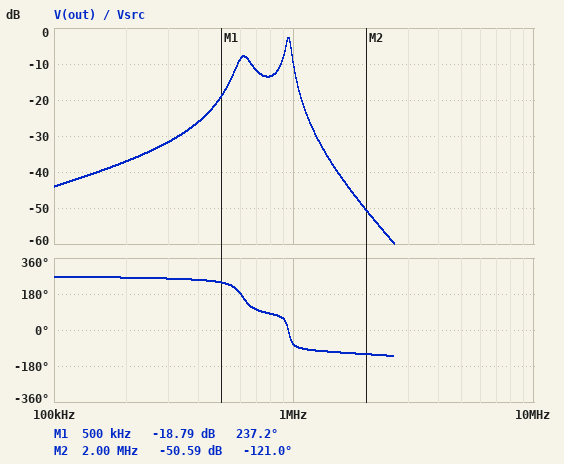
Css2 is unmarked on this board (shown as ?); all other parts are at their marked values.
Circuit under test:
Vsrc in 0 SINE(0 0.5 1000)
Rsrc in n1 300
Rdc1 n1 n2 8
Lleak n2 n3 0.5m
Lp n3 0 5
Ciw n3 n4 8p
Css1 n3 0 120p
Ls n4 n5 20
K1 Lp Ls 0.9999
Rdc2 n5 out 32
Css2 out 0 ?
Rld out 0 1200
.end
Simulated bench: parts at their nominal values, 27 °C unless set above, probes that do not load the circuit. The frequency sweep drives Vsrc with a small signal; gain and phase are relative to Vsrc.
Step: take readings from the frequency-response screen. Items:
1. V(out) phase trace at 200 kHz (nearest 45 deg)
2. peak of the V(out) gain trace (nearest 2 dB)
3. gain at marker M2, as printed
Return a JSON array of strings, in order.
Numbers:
["270 deg", "-2 dB", "-50.59 dB"]
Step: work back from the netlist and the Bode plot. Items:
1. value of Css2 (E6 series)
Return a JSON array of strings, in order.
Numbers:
["47 pF"]
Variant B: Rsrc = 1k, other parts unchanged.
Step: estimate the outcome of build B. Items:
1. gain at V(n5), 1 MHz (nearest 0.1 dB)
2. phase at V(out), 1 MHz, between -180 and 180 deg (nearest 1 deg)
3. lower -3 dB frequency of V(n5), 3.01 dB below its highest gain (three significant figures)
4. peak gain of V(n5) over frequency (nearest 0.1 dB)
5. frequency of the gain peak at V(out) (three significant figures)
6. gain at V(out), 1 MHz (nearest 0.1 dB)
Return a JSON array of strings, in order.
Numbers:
["-12.6 dB", "-52 deg", "907 kHz", "-5.6 dB", "943 kHz", "-12.9 dB"]
